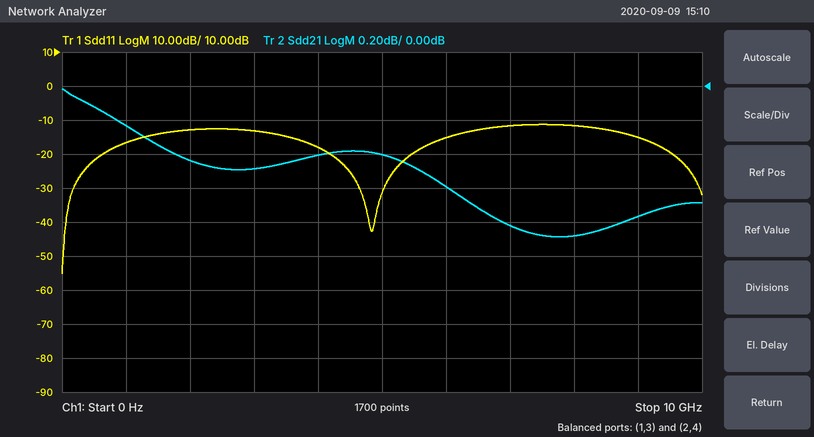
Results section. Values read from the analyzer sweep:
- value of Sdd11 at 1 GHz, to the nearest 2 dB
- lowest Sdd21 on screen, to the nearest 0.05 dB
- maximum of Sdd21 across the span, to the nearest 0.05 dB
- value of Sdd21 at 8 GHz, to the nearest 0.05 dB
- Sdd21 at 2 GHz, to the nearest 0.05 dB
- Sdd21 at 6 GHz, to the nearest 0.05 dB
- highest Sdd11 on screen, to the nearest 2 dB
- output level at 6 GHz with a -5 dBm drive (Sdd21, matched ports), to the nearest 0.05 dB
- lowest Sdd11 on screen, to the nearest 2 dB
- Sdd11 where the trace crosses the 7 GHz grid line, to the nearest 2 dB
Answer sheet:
-16 dB
-0.90 dB
0.00 dB
-0.90 dB
-0.45 dB
-0.60 dB
-12 dB
-5.60 dBm
-56 dB
-12 dB
